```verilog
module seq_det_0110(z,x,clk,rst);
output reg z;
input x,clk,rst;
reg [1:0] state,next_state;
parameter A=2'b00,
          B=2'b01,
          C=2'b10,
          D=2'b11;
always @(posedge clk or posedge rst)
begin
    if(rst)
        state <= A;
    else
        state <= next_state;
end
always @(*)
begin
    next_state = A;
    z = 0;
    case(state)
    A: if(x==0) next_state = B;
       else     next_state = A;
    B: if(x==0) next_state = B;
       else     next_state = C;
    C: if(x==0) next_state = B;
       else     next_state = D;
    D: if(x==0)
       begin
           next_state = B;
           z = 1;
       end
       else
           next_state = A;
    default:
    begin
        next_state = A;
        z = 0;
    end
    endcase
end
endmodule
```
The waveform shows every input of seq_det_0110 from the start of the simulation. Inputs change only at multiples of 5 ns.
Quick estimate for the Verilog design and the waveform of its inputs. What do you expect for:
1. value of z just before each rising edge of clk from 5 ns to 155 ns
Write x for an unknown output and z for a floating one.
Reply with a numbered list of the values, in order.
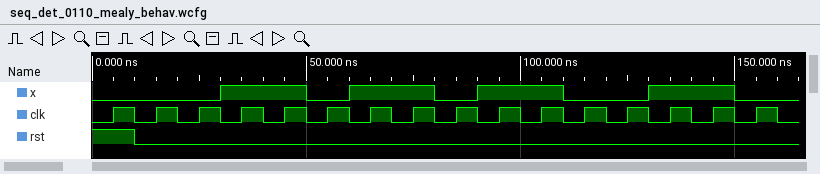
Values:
1. 0 0 0 0 0 1 0 0 1 0 0 1 0 0 0 1
